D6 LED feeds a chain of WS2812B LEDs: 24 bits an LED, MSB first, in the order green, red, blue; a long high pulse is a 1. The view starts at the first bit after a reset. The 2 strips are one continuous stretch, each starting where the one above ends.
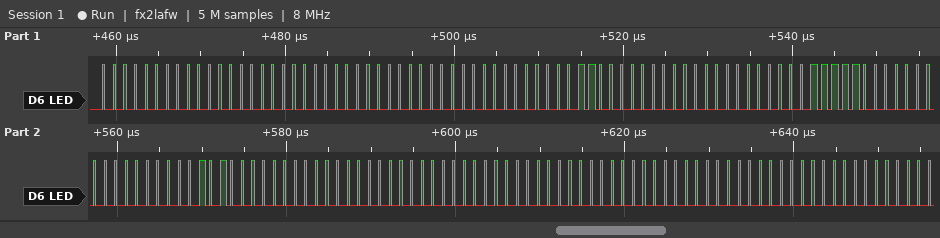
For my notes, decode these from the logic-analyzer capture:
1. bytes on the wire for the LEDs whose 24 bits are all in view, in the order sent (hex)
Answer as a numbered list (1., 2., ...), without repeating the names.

1. 00 00 00 00 00 06 00 00 1F 00 00 50 00 00 00 00 00 00
